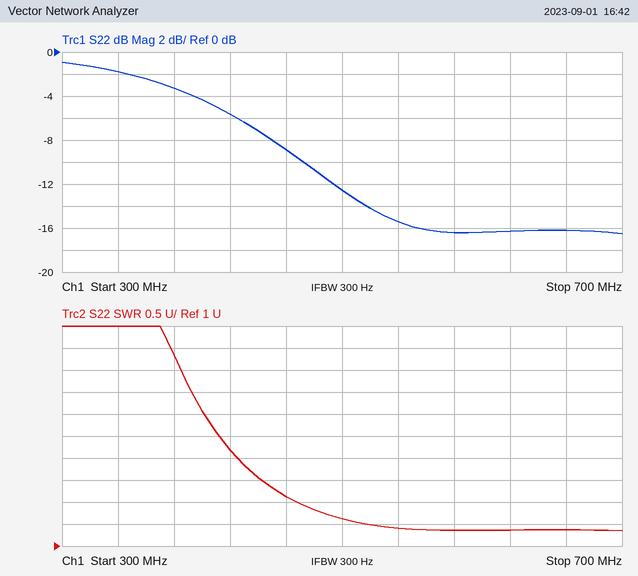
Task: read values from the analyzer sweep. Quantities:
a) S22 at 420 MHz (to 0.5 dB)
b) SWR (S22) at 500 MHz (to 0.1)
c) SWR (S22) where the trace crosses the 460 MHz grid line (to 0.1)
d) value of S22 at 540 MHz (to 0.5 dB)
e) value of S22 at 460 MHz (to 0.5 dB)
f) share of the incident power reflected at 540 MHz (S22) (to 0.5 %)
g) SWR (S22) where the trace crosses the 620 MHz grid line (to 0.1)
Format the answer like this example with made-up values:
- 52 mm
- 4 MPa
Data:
- -5.5 dB
- 1.6
- 2.1
- -15.5 dB
- -9.0 dB
- 3.0 %
- 1.4
